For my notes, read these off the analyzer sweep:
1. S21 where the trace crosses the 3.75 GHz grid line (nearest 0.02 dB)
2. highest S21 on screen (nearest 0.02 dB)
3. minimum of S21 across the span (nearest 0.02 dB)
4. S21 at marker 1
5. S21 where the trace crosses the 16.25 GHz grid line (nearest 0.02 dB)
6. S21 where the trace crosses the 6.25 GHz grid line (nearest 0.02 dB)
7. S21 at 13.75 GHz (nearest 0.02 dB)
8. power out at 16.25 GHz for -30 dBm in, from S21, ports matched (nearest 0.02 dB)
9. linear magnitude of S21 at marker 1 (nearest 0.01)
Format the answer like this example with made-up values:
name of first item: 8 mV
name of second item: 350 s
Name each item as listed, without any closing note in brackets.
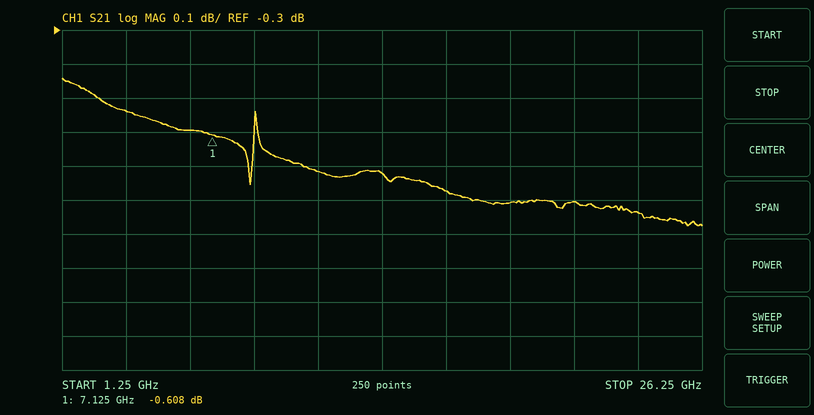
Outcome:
S21 where the trace crosses the 3.75 GHz grid line: -0.54 dB
highest S21 on screen: -0.44 dB
minimum of S21 across the span: -0.88 dB
S21 at marker 1: -0.608 dB
S21 where the trace crosses the 16.25 GHz grid line: -0.78 dB
S21 where the trace crosses the 6.25 GHz grid line: -0.60 dB
S21 at 13.75 GHz: -0.72 dB
power out at 16.25 GHz for -30 dBm in, from S21, ports matched: -30.78 dBm
linear magnitude of S21 at marker 1: 0.93
